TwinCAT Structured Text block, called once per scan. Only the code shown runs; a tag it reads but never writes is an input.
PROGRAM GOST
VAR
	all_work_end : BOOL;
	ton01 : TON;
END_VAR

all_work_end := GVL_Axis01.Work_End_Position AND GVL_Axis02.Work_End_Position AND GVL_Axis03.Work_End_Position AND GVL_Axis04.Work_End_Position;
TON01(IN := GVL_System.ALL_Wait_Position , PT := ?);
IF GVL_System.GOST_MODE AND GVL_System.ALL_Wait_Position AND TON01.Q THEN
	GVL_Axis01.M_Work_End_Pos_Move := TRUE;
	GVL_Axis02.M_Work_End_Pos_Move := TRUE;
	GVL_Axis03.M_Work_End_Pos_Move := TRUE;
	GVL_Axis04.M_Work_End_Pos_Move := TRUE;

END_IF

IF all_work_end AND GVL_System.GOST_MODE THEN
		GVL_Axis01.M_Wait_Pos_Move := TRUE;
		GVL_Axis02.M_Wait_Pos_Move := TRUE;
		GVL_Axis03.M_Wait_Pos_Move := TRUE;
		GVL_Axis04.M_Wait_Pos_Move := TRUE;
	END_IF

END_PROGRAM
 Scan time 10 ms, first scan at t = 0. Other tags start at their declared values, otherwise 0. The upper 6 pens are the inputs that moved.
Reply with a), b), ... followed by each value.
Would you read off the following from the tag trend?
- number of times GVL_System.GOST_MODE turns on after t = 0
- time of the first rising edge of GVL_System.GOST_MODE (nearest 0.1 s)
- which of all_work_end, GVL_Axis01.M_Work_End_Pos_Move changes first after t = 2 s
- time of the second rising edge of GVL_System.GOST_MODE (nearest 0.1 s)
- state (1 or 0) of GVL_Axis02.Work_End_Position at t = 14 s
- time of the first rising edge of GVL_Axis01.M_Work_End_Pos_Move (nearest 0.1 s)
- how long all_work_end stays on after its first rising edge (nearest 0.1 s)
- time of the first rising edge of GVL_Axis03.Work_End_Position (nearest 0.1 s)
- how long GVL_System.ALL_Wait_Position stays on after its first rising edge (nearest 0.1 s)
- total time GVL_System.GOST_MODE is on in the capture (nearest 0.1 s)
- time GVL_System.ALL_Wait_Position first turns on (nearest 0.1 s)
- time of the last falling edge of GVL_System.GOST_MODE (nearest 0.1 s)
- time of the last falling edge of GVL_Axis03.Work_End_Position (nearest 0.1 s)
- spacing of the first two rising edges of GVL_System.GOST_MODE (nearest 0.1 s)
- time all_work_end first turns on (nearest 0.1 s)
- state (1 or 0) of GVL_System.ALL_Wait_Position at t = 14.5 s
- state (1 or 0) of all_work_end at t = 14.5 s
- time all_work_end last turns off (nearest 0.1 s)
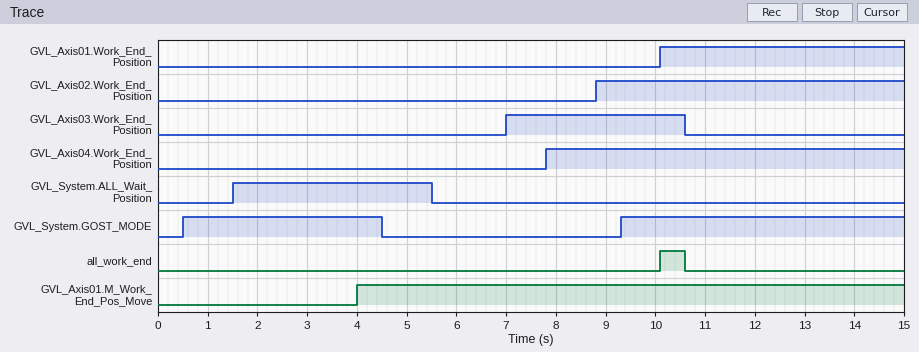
a) 2
b) 0.5 s
c) GVL_Axis01.M_Work_End_Pos_Move
d) 9.3 s
e) 1
f) 4.0 s
g) 0.5 s
h) 7.0 s
i) 4.0 s
j) 9.7 s
k) 1.5 s
l) 4.5 s
m) 10.6 s
n) 8.8 s
o) 10.1 s
p) 0
q) 0
r) 10.6 s
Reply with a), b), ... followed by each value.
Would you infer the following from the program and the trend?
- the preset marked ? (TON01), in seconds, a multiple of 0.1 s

a) 2.5 s
